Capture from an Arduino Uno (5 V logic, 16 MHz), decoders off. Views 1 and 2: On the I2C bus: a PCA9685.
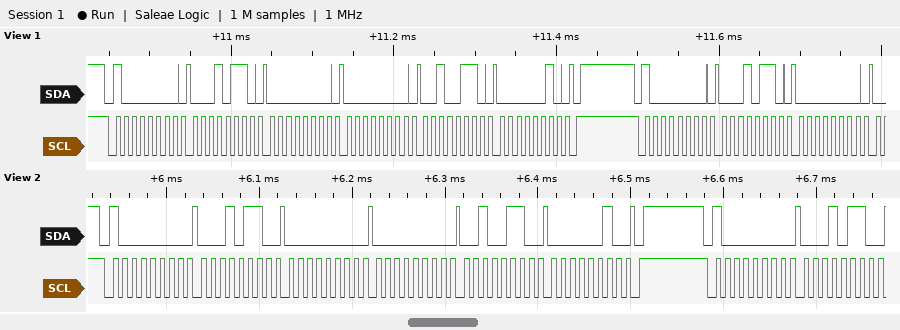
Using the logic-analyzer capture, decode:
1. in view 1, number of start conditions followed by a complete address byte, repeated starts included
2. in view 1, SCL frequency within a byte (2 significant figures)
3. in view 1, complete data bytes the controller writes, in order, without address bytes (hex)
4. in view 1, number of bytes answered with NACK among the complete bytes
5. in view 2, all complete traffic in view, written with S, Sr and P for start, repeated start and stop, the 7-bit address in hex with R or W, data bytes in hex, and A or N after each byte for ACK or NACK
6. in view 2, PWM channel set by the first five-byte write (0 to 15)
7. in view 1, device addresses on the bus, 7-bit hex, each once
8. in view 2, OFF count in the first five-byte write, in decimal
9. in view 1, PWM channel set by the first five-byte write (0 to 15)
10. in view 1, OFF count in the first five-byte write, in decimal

2
100 kHz
16 00 00 26 02 16 00
0
S 40W A 16 A 00 A 00 A 26 A 02 A P S 40W A 16 A
4
0x40
550
4
550
